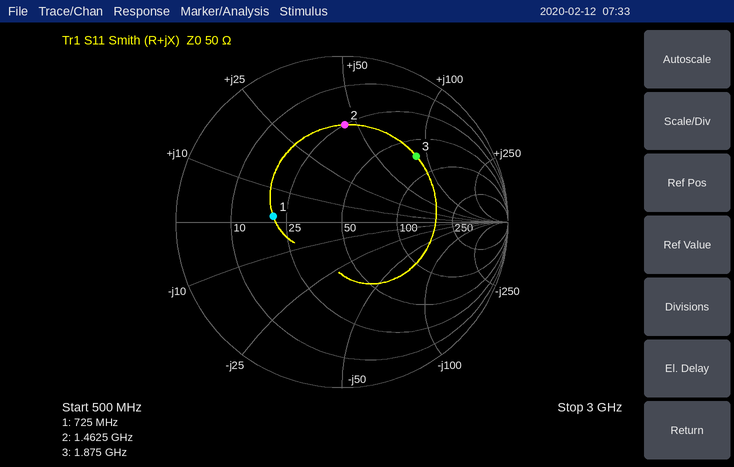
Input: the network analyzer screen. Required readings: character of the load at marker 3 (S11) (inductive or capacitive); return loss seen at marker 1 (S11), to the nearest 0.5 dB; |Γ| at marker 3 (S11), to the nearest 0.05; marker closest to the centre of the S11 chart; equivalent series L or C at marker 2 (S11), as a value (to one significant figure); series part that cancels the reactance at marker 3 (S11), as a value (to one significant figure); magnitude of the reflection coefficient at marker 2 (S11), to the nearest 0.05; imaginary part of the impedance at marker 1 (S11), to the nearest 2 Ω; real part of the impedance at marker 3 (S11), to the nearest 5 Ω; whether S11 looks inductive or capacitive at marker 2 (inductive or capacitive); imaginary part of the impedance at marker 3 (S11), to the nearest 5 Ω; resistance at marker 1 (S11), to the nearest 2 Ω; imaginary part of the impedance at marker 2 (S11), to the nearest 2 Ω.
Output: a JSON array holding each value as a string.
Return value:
["inductive", "7.5 dB", "0.60", "marker 1", "5 nH", "1.0 pF", "0.60", "+2 Ω", "70 Ω", "inductive", "+85 Ω", "20 Ω", "+44 Ω"]
